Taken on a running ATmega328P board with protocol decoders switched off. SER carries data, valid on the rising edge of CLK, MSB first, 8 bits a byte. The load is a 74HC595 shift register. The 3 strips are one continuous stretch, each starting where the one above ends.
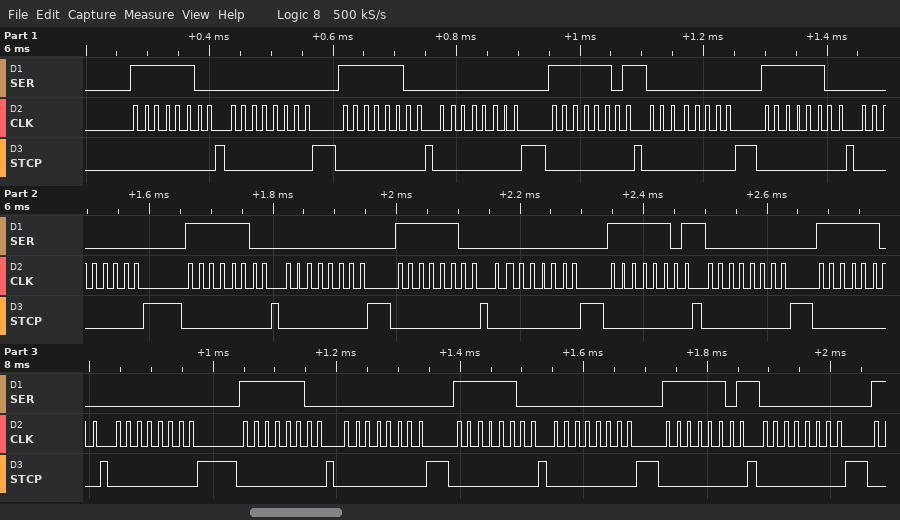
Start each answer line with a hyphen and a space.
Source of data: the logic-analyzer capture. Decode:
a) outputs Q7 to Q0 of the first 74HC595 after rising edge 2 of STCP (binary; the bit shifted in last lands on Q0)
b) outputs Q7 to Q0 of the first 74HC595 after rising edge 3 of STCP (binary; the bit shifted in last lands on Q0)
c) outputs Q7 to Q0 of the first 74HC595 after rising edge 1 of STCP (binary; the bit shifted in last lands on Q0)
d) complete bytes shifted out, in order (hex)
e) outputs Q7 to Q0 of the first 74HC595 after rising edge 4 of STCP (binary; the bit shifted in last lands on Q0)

- 00000000
- 11111100
- 11111100
- FC 00 FC 00 FD 00 FC 00 FC 00 FC 00 FD 00 FC 00 FC 00 FC 00 FD 00
- 00000000
